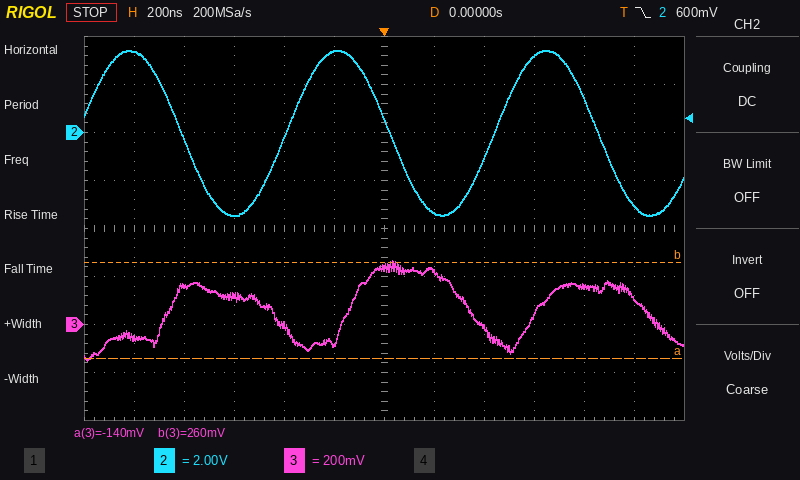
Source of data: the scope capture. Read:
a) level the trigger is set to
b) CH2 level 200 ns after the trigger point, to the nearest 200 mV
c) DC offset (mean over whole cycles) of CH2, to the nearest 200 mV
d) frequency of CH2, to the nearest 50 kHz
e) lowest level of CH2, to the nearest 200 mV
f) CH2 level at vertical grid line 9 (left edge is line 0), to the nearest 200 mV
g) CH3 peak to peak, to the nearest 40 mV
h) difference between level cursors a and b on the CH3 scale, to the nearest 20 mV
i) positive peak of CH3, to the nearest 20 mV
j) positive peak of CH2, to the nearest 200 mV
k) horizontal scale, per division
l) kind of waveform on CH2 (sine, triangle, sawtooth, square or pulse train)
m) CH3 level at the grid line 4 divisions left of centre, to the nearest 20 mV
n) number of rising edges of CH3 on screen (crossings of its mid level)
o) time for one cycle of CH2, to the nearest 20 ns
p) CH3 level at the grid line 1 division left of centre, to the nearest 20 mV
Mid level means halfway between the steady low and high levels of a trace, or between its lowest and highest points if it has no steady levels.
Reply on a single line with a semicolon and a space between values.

600 mV; -3.4 V; 0.0 V; 1.20 MHz; -3.4 V; 3.2 V; 400 mV; 400 mV; 260 mV; 3.4 V; 200 ns; sine; 160 mV; 3; 840 ns; -80 mV
